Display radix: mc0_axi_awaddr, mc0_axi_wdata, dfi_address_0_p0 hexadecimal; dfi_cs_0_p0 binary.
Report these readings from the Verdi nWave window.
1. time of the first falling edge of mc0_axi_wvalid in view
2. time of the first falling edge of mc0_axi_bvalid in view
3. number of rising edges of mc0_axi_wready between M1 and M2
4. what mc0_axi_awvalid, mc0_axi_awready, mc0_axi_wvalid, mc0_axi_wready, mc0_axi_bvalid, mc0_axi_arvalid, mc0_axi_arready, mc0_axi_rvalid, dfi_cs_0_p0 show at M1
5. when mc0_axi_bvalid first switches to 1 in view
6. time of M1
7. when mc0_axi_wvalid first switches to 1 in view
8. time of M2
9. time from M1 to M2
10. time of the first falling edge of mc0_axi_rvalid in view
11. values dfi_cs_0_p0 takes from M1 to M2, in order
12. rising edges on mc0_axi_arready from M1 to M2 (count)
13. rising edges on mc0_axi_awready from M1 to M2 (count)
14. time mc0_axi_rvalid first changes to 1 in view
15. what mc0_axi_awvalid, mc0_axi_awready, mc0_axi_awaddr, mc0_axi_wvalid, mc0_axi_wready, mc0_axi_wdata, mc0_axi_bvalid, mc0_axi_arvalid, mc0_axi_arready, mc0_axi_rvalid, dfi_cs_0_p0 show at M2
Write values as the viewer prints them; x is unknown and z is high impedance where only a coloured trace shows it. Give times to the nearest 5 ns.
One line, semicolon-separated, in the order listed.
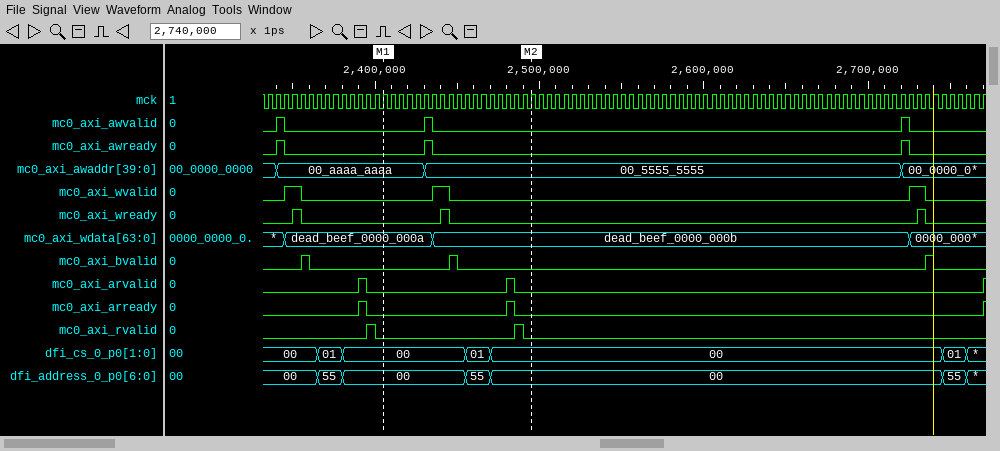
2355 ns; 2360 ns; 1; mc0_axi_awvalid=0, mc0_axi_awready=0, mc0_axi_wvalid=0, mc0_axi_wready=0, mc0_axi_bvalid=0, mc0_axi_arvalid=0, mc0_axi_arready=0, mc0_axi_rvalid=0, dfi_cs_0_p0=00; 2355 ns; 2405 ns; 2345 ns; 2495 ns; 90 ns; 2400 ns; 00, 01, 00; 1; 1; 2395 ns; mc0_axi_awvalid=0, mc0_axi_awready=0, mc0_axi_awaddr=00_5555_5555, mc0_axi_wvalid=0, mc0_axi_wready=0, mc0_axi_wdata=dead_beef_0000_000b, mc0_axi_bvalid=0, mc0_axi_arvalid=0, mc0_axi_arready=0, mc0_axi_rvalid=0, dfi_cs_0_p0=00
